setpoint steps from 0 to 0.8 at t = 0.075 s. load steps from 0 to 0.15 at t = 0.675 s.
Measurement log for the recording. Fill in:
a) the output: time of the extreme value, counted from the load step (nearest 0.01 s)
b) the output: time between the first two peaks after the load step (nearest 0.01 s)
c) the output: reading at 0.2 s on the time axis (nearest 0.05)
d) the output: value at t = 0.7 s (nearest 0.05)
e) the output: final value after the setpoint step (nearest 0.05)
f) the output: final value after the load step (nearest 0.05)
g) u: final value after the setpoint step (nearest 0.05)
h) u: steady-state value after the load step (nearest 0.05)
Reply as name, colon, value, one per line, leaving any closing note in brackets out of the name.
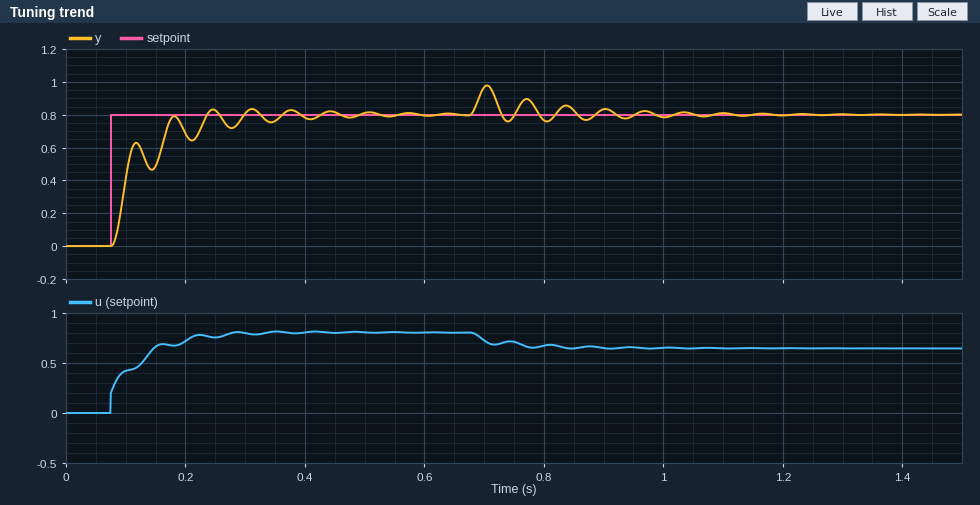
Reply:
the output: time of the extreme value, counted from the load step: 0.03 s
the output: time between the first two peaks after the load step: 0.07 s
the output: reading at 0.2 s on the time axis: 0.70
the output: value at t = 0.7 s: 0.95
the output: final value after the setpoint step: 0.80
the output: final value after the load step: 0.80
u: final value after the setpoint step: 0.80
u: steady-state value after the load step: 0.65
